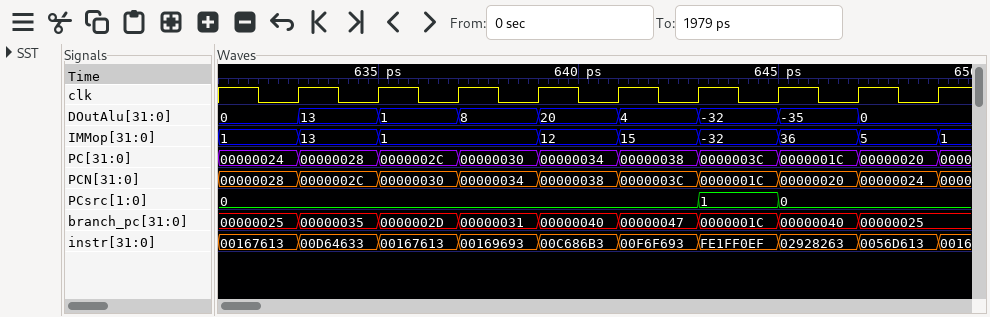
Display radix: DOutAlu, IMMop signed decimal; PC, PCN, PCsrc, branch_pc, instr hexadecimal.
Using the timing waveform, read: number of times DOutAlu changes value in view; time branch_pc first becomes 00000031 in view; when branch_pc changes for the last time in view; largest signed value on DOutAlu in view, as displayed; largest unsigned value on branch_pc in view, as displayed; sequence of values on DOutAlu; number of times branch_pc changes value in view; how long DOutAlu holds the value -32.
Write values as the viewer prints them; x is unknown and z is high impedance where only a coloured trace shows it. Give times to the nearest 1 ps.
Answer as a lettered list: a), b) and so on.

a) 8
b) 637 ps
c) 647 ps
d) 20
e) 00000047
f) 0, 13, 1, 8, 20, 4, -32, -35, 0
g) 8
h) 2 ps
